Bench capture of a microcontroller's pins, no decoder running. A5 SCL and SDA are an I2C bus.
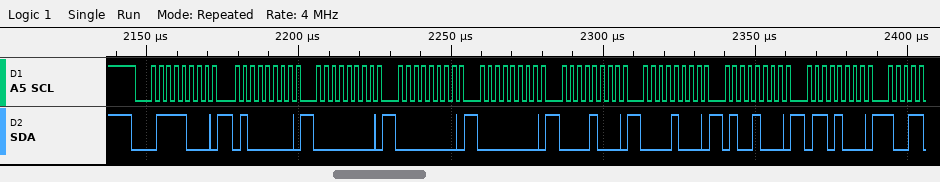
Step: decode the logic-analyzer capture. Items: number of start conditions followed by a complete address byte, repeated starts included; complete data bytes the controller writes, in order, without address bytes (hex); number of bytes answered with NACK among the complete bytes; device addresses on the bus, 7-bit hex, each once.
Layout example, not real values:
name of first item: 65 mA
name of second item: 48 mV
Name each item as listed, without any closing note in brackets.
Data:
number of start conditions followed by a complete address byte, repeated starts included: 1
complete data bytes the controller writes, in order, without address bytes: 40 00 00 00 08 08 48 68
number of bytes answered with NACK among the complete bytes: 0
device addresses on the bus, 7-bit hex, each once: 0x3C
